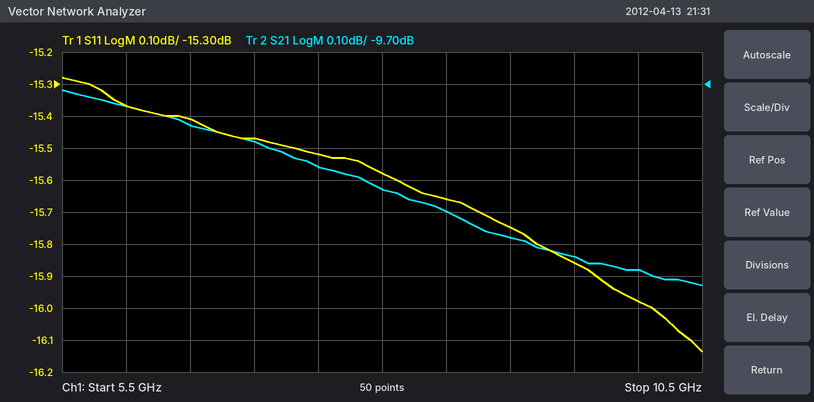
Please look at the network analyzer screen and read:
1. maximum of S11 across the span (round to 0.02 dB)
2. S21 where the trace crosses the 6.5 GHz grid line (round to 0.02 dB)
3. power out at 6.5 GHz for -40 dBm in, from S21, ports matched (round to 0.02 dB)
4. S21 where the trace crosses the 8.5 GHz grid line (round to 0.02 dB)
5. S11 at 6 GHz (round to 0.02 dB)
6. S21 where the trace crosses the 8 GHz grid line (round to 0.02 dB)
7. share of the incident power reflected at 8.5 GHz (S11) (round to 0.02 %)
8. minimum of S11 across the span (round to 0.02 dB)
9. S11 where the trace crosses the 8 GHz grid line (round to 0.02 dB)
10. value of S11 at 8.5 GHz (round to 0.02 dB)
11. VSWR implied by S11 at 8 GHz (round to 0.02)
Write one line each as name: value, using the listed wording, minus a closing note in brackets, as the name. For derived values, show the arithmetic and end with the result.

maximum of S11 across the span: -15.28 dB
S21 where the trace crosses the 6.5 GHz grid line: -9.82 dB
power out at 6.5 GHz for -40 dBm in, from S21, ports matched: -40 dBm + (-9.82 dB) = -49.82 dBm
S21 where the trace crosses the 8.5 GHz grid line: -10.10 dB
S11 at 6 GHz: -15.36 dB
S21 where the trace crosses the 8 GHz grid line: -10.02 dB
share of the incident power reflected at 8.5 GHz (S11): 10^(-15.66/10) ≈ 2.72 %
minimum of S11 across the span: -16.14 dB
S11 where the trace crosses the 8 GHz grid line: -15.58 dB
value of S11 at 8.5 GHz: -15.66 dB
VSWR implied by S11 at 8 GHz: |Γ| = 10^(-15.58/20) = 0.1663; VSWR = (1 + 0.1663)/(1 − 0.1663) ≈ 1.40
